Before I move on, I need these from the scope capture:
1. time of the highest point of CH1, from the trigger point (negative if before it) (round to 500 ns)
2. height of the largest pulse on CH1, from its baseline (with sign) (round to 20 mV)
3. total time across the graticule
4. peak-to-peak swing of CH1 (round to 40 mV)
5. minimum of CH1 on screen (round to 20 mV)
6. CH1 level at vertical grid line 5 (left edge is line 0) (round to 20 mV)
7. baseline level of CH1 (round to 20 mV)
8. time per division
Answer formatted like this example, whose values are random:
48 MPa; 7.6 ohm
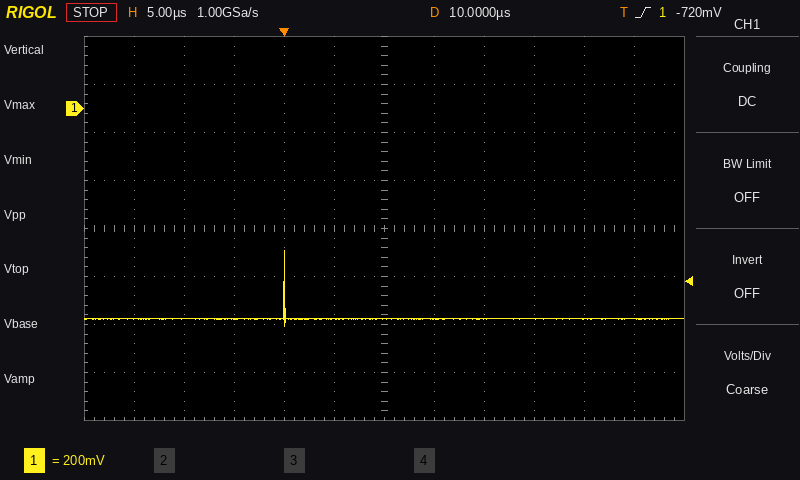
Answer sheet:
0.0 µs; +280 mV; 60 µs; 320 mV; -900 mV; -880 mV; -880 mV; 5 µs
